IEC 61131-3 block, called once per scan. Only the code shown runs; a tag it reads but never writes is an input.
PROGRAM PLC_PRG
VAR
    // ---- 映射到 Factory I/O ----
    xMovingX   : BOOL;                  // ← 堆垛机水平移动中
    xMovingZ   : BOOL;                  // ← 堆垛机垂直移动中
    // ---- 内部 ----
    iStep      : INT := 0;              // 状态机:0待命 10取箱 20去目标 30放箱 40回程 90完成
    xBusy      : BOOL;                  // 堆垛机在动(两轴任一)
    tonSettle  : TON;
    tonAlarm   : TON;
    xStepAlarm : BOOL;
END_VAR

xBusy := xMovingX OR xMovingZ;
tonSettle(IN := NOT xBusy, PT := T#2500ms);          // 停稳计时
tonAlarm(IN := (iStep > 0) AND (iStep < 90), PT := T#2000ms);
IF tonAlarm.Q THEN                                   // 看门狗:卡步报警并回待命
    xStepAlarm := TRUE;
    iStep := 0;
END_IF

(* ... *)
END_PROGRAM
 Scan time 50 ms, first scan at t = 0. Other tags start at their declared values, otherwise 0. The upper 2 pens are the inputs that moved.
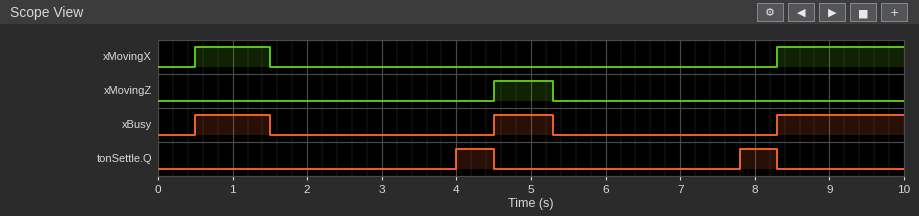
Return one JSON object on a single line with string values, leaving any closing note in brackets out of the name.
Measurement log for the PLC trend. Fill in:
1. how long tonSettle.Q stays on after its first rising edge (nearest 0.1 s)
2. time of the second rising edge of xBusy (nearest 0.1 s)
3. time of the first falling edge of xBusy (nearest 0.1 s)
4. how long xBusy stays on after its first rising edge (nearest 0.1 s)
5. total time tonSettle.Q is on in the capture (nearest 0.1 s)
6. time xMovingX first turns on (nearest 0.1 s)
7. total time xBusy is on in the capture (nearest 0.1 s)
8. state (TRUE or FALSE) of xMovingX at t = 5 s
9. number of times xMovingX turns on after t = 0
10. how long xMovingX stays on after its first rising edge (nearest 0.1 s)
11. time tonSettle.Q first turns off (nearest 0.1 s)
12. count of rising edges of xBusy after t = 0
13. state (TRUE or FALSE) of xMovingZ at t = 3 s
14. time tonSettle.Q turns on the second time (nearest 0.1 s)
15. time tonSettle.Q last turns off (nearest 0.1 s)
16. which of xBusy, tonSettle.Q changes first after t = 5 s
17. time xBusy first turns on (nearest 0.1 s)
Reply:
{"how long tonSettle.Q stays on after its first rising edge": "0.5 s", "time of the second rising edge of xBusy": "4.5 s", "time of the first falling edge of xBusy": "1.5 s", "how long xBusy stays on after its first rising edge": "1.0 s", "total time tonSettle.Q is on in the capture": "1.0 s", "time xMovingX first turns on": "0.5 s", "total time xBusy is on in the capture": "3.5 s", "state (TRUE or FALSE) of xMovingX at t = 5 s": "FALSE", "number of times xMovingX turns on after t = 0": "2", "how long xMovingX stays on after its first rising edge": "1.0 s", "time tonSettle.Q first turns off": "4.5 s", "count of rising edges of xBusy after t = 0": "3", "state (TRUE or FALSE) of xMovingZ at t = 3 s": "FALSE", "time tonSettle.Q turns on the second time": "7.8 s", "time tonSettle.Q last turns off": "8.3 s", "which of xBusy, tonSettle.Q changes first after t = 5 s": "xBusy", "time xBusy first turns on": "0.5 s"}
